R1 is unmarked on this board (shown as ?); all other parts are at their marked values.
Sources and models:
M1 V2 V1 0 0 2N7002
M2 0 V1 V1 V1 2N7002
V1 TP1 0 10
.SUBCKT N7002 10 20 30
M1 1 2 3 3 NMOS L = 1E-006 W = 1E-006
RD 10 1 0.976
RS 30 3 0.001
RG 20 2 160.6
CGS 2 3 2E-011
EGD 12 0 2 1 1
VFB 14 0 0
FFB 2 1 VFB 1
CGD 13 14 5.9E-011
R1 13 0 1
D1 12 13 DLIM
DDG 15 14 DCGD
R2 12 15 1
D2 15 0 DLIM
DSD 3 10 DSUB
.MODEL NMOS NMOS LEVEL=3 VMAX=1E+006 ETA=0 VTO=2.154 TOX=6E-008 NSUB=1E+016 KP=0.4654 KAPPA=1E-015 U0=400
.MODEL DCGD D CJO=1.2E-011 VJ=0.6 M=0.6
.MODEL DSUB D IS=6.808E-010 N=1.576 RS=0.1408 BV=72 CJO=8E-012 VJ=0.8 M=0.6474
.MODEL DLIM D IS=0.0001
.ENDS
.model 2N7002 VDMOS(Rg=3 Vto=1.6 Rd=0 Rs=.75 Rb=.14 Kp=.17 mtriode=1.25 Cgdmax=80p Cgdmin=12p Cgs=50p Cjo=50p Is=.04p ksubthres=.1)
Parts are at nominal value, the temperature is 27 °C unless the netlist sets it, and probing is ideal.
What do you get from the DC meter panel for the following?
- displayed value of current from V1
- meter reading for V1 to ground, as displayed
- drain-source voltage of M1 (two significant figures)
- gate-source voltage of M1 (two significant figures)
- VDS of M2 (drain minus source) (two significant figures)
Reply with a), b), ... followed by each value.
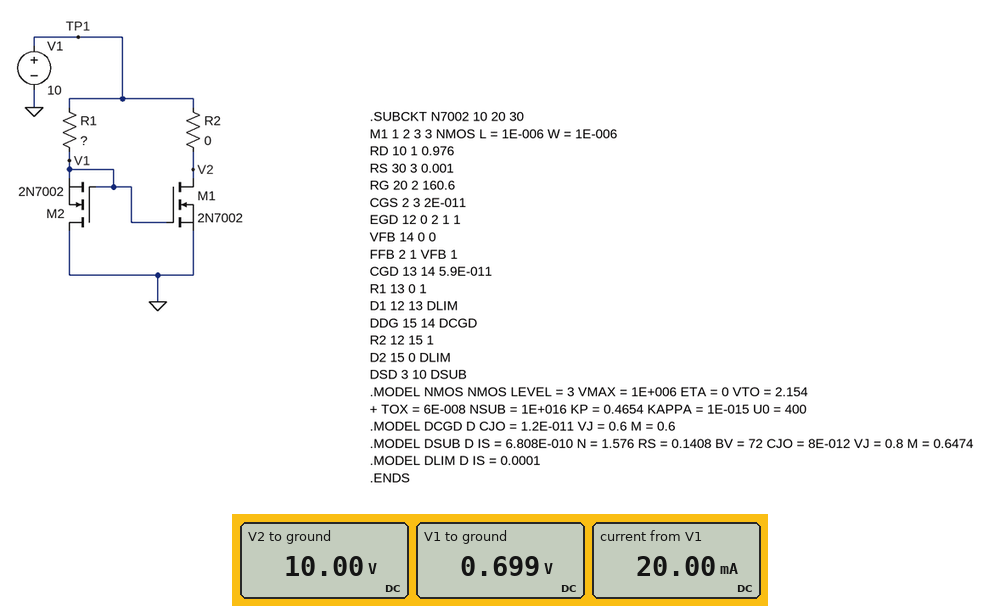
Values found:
a) 20.00 mA
b) 0.699 V
c) 10 V
d) 700 mV
e) -700 mV
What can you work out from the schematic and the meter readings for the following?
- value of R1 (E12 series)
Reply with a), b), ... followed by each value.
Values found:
a) 470 Ω
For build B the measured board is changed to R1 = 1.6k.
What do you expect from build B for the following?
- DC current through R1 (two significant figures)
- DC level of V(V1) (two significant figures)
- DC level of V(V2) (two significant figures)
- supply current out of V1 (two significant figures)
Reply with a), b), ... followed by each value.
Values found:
a) 5.8 mA
b) 670 mV
c) 10 V
d) 5.4 mA
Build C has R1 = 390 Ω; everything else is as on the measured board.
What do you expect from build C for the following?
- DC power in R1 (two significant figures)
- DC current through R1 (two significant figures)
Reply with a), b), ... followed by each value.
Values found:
a) 220 mW
b) 24 mA
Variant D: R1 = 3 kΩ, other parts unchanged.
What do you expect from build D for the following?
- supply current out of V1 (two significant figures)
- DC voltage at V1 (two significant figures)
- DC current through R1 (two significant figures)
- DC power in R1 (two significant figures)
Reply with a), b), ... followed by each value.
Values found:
a) 3.7 mA
b) 650 mV
c) 3.1 mA
d) 29 mW
